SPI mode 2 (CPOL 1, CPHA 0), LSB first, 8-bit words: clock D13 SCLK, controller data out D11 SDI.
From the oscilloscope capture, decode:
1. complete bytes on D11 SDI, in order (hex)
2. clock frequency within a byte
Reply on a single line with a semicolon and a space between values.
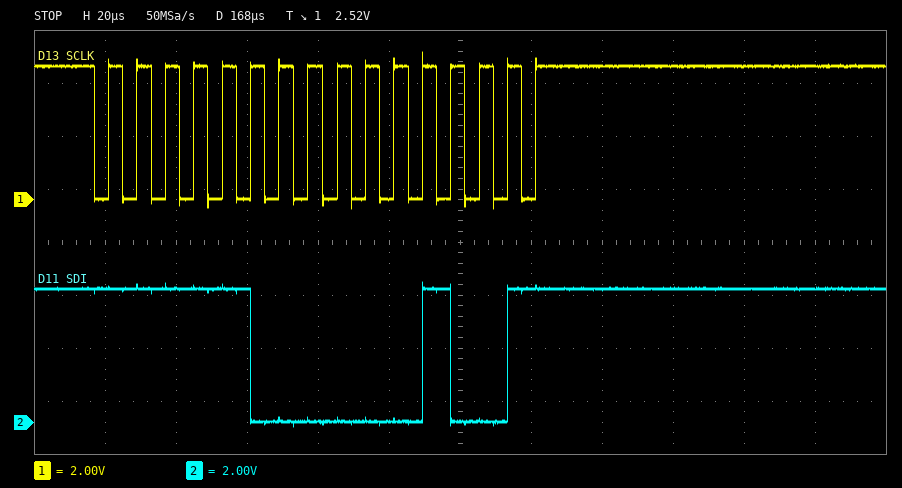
3F 90; 125 kHz
